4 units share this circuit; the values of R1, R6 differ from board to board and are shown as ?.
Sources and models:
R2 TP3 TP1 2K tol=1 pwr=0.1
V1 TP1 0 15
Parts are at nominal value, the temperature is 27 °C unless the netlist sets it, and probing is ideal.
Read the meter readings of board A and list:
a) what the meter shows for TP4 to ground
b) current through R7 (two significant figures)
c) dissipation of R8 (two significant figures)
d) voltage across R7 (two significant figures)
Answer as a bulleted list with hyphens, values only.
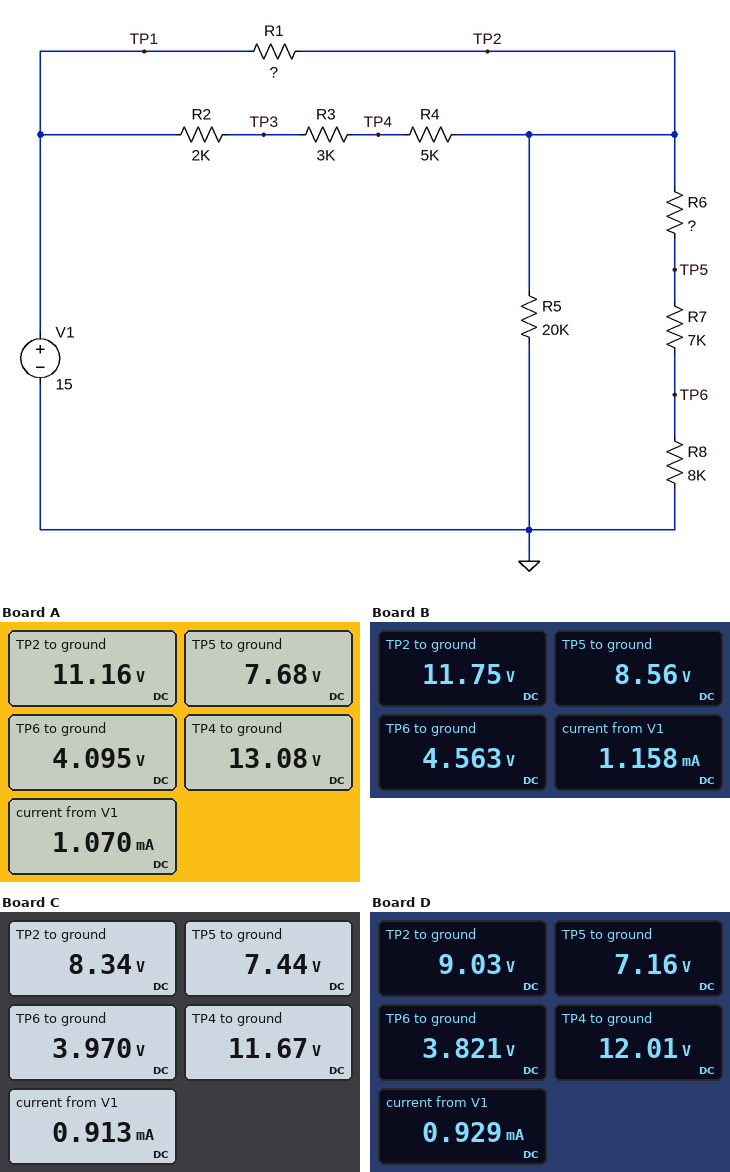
- 13.08 V
- 510 µA
- 2.1 mW
- 3.6 V
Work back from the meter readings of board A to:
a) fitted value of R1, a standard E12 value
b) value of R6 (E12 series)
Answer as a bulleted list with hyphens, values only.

- 5.6 kΩ
- 6.8 kΩ
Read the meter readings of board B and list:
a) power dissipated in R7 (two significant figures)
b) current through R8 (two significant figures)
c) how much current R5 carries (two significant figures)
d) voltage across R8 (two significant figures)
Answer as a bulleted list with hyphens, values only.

- 2.3 mW
- 570 µA
- 590 µA
- 4.6 V
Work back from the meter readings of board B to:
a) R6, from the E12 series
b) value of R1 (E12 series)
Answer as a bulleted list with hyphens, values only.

- 5.6 kΩ
- 3.9 kΩ
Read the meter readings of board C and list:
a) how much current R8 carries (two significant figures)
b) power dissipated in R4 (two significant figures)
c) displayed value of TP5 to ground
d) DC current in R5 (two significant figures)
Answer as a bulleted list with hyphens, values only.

- 500 µA
- 2.2 mW
- 7.44 V
- 420 µA
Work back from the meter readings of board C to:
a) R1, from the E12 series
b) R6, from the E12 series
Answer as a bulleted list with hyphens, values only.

- 27 kΩ
- 1.8 kΩ
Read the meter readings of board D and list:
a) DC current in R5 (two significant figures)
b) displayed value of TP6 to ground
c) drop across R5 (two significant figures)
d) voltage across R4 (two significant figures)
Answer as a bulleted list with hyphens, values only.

- 450 µA
- 3.821 V
- 9.0 V
- 3.0 V
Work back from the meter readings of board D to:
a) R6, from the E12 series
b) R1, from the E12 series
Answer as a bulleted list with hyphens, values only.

- 3.9 kΩ
- 18 kΩ
